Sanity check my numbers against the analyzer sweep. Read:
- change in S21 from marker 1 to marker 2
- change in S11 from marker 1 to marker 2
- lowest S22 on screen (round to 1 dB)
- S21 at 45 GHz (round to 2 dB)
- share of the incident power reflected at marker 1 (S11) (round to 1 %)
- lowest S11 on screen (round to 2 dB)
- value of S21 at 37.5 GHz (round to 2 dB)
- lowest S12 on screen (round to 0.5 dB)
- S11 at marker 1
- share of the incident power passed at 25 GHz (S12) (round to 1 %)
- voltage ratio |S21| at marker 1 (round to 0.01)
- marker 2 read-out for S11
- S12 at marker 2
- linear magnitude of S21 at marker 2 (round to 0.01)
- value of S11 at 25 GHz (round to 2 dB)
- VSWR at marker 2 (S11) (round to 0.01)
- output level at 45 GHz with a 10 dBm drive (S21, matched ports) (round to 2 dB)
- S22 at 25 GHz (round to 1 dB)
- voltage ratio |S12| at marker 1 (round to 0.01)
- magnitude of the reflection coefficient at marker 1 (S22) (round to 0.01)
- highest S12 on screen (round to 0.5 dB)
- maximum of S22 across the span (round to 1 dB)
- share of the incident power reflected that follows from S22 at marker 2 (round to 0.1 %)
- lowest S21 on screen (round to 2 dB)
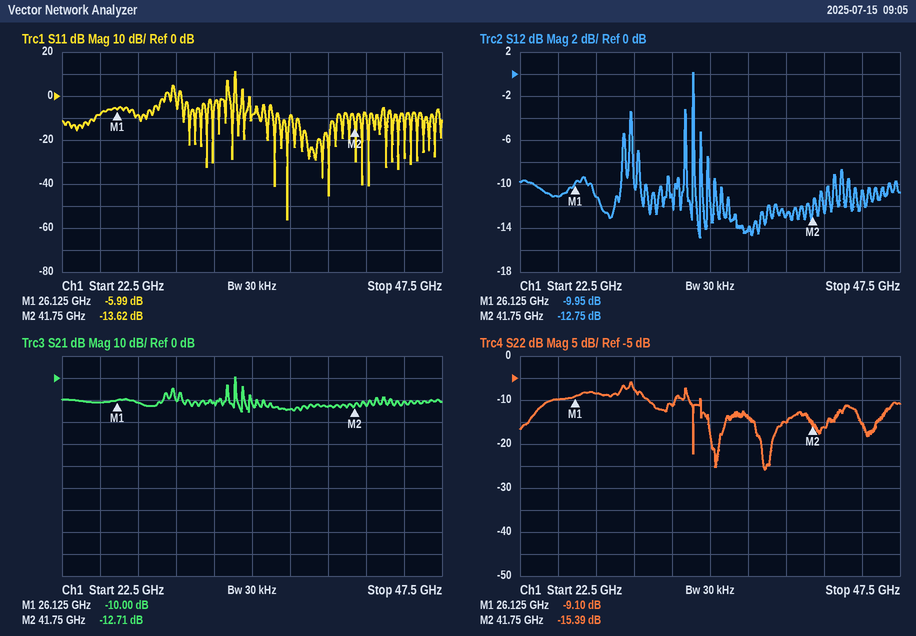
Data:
-2.71 dB
-7.63 dB
-26 dB
-10 dB
25 %
-56 dB
-14 dB
-15.0 dB
-5.99 dB
8 %
0.32
-13.62 dB
-12.75 dB
0.23
-8 dB
1.53
0 dBm
-10 dB
0.32
0.35
0.0 dB
-6 dB
2.9 %
-16 dB
